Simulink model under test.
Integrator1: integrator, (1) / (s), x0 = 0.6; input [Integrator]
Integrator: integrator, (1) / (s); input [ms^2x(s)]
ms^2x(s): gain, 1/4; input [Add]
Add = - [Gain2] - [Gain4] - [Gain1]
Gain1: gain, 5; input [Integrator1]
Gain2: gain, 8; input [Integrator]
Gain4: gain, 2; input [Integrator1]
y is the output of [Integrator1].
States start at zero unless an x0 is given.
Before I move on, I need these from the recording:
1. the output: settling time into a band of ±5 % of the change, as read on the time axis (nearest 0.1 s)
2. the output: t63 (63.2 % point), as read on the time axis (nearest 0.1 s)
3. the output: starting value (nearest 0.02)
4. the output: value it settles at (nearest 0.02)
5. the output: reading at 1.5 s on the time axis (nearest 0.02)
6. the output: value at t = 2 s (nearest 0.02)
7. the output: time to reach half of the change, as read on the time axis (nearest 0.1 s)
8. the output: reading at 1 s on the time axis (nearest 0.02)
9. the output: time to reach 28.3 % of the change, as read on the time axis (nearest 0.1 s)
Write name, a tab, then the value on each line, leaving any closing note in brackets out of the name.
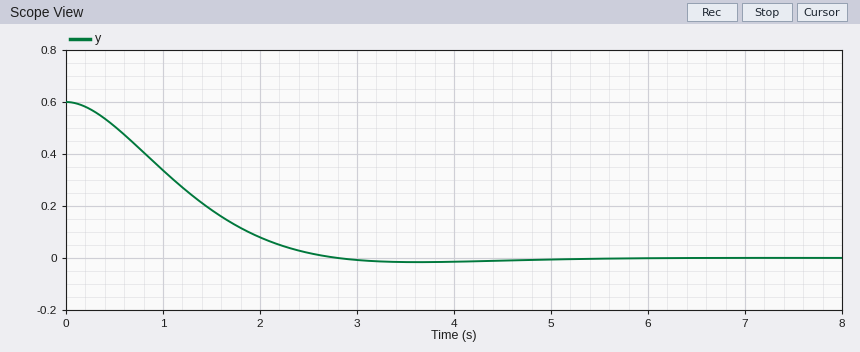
the output: settling time into a band of ±5 % of the change, as read on the time axis	2.4 s
the output: t63 (63.2 % point), as read on the time axis	1.4 s
the output: starting value	0.60
the output: value it settles at	0.00
the output: reading at 1.5 s on the time axis	0.18
the output: value at t = 2 s	0.08
the output: time to reach half of the change, as read on the time axis	1.1 s
the output: reading at 1 s on the time axis	0.34
the output: time to reach 28.3 % of the change, as read on the time axis	0.7 s
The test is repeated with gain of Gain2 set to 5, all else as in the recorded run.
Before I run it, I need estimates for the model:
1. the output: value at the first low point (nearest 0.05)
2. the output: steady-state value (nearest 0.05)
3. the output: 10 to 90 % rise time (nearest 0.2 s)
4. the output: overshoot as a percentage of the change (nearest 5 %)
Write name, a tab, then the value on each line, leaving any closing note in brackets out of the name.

the output: value at the first low point	-0.10
the output: steady-state value	0.00
the output: 10 to 90 % rise time	1.2 s
the output: overshoot as a percentage of the change	20 %
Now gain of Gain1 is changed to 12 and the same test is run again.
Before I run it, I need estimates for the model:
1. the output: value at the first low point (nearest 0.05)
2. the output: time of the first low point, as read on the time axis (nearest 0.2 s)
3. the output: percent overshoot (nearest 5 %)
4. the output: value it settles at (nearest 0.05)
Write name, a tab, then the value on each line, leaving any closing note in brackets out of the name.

the output: value at the first low point	-0.10
the output: time of the first low point, as read on the time axis	2.0 s
the output: percent overshoot	15 %
the output: value it settles at	0.00
